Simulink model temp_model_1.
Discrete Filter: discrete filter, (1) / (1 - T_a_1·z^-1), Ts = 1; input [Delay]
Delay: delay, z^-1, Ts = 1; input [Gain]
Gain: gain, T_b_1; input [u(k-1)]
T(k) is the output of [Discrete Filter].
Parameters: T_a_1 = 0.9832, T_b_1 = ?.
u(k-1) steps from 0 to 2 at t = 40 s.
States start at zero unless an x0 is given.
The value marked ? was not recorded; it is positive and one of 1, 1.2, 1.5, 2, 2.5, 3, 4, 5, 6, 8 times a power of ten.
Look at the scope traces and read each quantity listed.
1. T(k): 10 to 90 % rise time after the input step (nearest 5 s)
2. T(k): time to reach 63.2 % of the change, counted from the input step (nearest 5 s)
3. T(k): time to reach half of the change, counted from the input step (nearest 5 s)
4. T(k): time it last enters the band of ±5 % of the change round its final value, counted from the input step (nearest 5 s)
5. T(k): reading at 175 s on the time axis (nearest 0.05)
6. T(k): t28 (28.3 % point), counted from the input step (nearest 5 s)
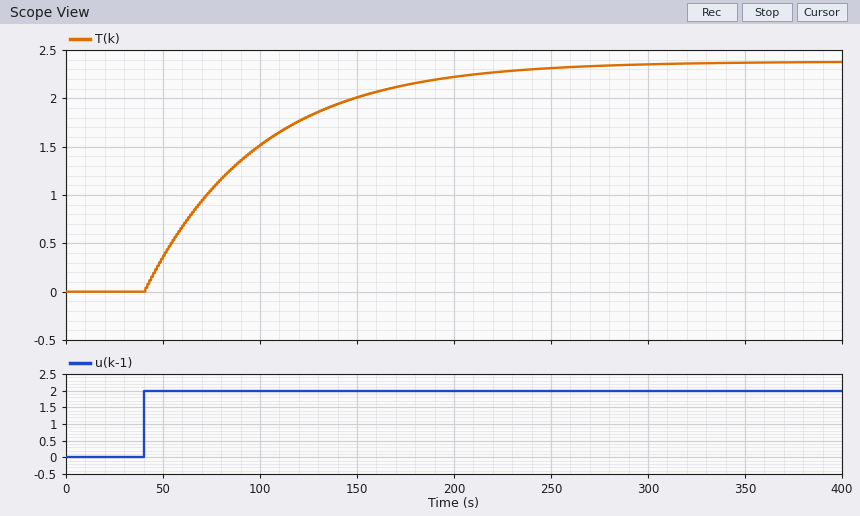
130 s
60 s
40 s
175 s
2.15
20 s
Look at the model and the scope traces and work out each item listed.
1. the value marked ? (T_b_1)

0.02
